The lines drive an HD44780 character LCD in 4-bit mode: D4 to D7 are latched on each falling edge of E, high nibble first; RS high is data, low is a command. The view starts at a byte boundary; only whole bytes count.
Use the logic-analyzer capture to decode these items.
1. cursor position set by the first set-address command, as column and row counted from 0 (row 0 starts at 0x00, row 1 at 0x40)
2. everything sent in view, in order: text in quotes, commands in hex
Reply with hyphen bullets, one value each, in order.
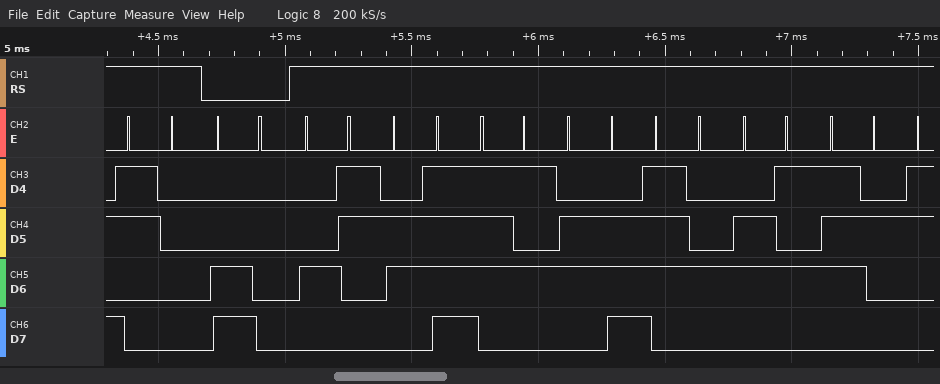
- column 0, row 1
- "0" 0xC0 "Counter"
